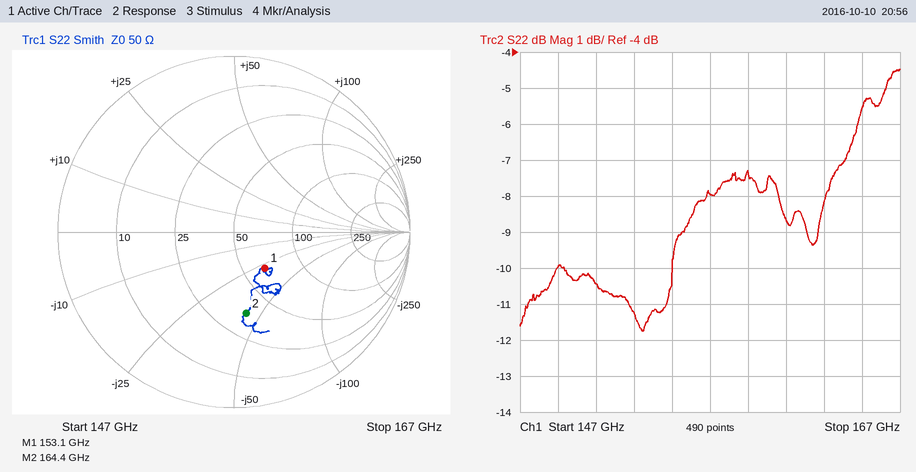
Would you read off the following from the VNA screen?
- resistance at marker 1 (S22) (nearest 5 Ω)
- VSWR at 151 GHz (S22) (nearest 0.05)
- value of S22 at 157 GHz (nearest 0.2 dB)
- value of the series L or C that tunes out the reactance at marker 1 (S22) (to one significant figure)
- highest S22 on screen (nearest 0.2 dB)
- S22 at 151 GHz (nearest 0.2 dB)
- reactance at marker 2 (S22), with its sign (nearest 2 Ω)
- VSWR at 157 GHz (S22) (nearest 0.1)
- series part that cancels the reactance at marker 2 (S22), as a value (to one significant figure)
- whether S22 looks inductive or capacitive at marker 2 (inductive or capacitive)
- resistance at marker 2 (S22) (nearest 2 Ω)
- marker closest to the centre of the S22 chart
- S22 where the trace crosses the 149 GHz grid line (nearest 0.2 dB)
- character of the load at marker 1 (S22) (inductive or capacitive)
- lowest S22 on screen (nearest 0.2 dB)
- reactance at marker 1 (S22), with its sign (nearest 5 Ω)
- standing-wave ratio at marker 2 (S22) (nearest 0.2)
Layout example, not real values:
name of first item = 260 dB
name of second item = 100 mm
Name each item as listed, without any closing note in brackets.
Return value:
resistance at marker 1 (S22) = 65 Ω
VSWR at 151 GHz (S22) = 1.85
value of S22 at 157 GHz = -8.0 dB
value of the series L or C that tunes out the reactance at marker 1 (S22) = 30 pH
highest S22 on screen = -4.4 dB
S22 at 151 GHz = -10.4 dB
reactance at marker 2 (S22), with its sign = -42 Ω
VSWR at 157 GHz (S22) = 2.3
series part that cancels the reactance at marker 2 (S22), as a value = 40 pH
whether S22 looks inductive or capacitive at marker 2 = capacitive
resistance at marker 2 (S22) = 36 Ω
marker closest to the centre of the S22 chart = marker 1
S22 where the trace crosses the 149 GHz grid line = -10.0 dB
character of the load at marker 1 (S22) = capacitive
lowest S22 on screen = -11.8 dB
reactance at marker 1 (S22), with its sign = -30 Ω
standing-wave ratio at marker 2 (S22) = 2.8
